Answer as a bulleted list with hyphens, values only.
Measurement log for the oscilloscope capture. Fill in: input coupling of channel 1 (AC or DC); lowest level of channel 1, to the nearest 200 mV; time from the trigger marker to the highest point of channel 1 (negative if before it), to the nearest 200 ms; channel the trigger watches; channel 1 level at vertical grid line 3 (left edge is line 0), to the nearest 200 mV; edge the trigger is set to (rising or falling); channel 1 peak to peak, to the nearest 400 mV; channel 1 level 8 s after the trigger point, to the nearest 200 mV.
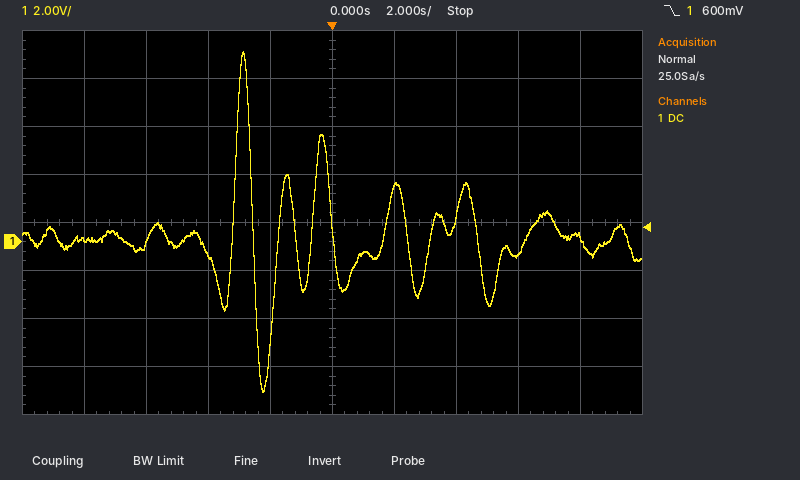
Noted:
- DC
- -6.2 V
- -2.8 s
- channel 1
- -600 mV
- falling
- 14.0 V
- 200 mV
